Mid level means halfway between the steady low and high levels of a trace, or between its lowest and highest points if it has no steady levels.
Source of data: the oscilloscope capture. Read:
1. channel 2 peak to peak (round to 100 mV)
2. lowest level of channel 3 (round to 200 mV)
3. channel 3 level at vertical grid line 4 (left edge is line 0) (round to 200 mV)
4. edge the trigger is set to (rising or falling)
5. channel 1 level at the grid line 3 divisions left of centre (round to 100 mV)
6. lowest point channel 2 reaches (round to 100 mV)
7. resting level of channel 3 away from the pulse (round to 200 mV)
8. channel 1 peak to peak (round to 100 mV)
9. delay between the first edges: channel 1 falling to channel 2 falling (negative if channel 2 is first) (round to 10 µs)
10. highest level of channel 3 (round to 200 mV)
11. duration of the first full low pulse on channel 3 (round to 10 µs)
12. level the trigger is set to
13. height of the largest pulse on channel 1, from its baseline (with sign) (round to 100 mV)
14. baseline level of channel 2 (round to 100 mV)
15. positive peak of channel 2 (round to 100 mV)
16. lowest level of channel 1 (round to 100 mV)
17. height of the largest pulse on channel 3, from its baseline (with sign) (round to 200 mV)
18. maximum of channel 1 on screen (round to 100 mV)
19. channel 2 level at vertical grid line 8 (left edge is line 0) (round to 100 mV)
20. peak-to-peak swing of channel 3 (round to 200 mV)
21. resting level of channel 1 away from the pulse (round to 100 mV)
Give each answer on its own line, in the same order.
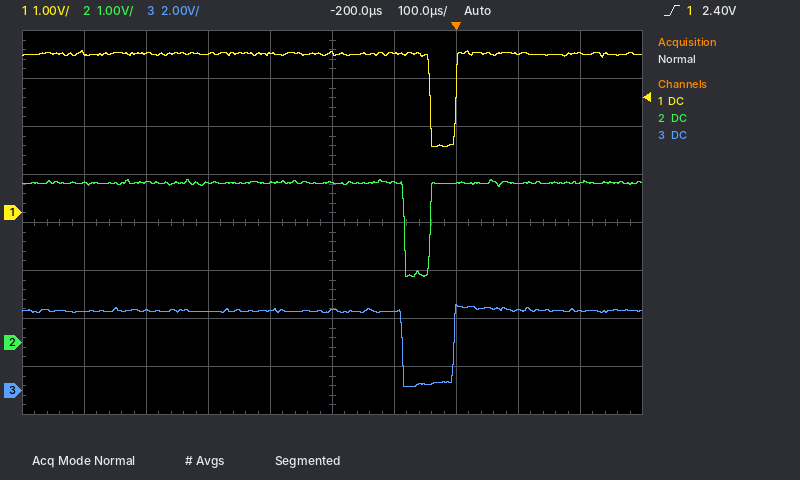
2.0 V
200 mV
3.4 V
rising
3.3 V
1.4 V
3.4 V
2.0 V
-40 µs
3.6 V
80 µs
2.40 V
-1.9 V
3.3 V
3.4 V
1.4 V
-3.2 V
3.4 V
3.3 V
3.4 V
3.3 V
